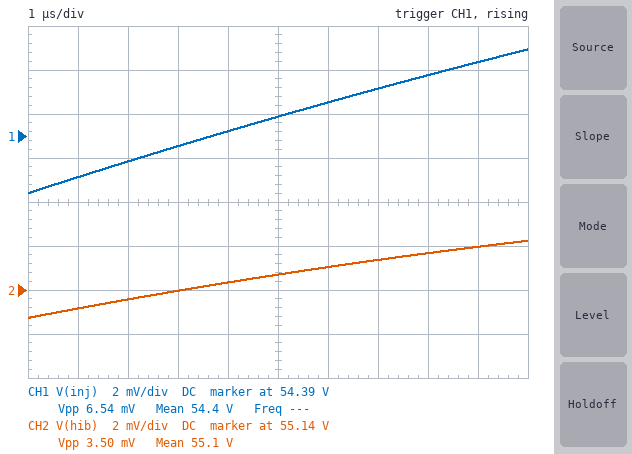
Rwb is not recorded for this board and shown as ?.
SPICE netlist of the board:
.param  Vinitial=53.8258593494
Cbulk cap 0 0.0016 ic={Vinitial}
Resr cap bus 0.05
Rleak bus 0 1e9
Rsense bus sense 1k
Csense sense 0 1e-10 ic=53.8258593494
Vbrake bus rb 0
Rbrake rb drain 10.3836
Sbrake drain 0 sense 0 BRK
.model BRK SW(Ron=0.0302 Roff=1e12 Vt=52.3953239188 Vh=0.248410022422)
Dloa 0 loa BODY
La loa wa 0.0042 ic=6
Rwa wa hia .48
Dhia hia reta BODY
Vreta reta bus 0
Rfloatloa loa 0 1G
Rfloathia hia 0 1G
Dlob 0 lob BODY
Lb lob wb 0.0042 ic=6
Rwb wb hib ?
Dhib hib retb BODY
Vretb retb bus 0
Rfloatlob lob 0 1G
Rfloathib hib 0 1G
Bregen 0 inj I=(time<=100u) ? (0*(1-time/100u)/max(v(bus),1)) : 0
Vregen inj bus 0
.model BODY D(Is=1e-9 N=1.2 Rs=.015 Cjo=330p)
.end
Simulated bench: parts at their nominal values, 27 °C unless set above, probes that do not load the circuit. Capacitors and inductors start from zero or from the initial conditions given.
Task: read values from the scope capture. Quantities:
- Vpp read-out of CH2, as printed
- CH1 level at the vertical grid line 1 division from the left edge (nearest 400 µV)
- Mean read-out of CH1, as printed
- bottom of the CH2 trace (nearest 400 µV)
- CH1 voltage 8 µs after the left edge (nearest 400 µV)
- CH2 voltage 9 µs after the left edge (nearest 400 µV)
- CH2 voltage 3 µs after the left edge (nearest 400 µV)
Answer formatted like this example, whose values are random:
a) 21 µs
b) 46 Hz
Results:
a) 3.50 mV
b) 54.3880 V
c) 54.4 V
d) 55.1408 V
e) 54.3928 V
f) 55.1440 V
g) 55.1420 V
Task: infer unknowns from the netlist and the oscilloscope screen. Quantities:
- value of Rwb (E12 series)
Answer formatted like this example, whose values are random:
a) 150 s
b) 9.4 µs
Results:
a) 0.27 Ω
